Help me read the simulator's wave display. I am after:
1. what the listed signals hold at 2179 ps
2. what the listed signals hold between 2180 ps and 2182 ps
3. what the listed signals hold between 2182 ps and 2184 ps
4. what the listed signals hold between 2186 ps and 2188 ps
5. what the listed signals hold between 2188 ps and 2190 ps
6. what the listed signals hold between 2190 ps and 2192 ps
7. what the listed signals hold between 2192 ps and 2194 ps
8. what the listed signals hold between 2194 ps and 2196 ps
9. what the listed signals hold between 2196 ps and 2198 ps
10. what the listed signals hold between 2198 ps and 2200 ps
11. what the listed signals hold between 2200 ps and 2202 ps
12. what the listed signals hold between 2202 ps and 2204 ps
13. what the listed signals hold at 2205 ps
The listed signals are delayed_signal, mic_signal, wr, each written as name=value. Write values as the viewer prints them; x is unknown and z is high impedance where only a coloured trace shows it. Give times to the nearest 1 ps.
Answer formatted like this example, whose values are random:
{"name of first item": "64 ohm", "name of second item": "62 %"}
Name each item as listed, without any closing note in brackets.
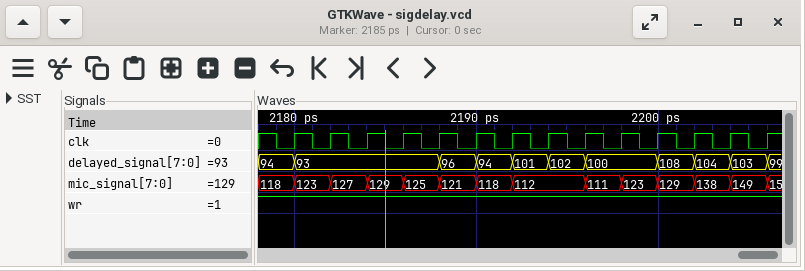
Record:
{"what the listed signals hold at 2179 ps": "delayed_signal=94, mic_signal=118, wr=1", "what the listed signals hold between 2180 ps and 2182 ps": "delayed_signal=93, mic_signal=123, wr=1", "what the listed signals hold between 2182 ps and 2184 ps": "delayed_signal=93, mic_signal=127, wr=1", "what the listed signals hold between 2186 ps and 2188 ps": "delayed_signal=93, mic_signal=125, wr=1", "what the listed signals hold between 2188 ps and 2190 ps": "delayed_signal=96, mic_signal=121, wr=1", "what the listed signals hold between 2190 ps and 2192 ps": "delayed_signal=94, mic_signal=118, wr=1", "what the listed signals hold between 2192 ps and 2194 ps": "delayed_signal=101, mic_signal=112, wr=1", "what the listed signals hold between 2194 ps and 2196 ps": "delayed_signal=102, mic_signal=112, wr=1", "what the listed signals hold between 2196 ps and 2198 ps": "delayed_signal=100, mic_signal=111, wr=1", "what the listed signals hold between 2198 ps and 2200 ps": "delayed_signal=100, mic_signal=123, wr=1", "what the listed signals hold between 2200 ps and 2202 ps": "delayed_signal=108, mic_signal=129, wr=1", "what the listed signals hold between 2202 ps and 2204 ps": "delayed_signal=104, mic_signal=138, wr=1", "what the listed signals hold at 2205 ps": "delayed_signal=103, mic_signal=149, wr=1"}
